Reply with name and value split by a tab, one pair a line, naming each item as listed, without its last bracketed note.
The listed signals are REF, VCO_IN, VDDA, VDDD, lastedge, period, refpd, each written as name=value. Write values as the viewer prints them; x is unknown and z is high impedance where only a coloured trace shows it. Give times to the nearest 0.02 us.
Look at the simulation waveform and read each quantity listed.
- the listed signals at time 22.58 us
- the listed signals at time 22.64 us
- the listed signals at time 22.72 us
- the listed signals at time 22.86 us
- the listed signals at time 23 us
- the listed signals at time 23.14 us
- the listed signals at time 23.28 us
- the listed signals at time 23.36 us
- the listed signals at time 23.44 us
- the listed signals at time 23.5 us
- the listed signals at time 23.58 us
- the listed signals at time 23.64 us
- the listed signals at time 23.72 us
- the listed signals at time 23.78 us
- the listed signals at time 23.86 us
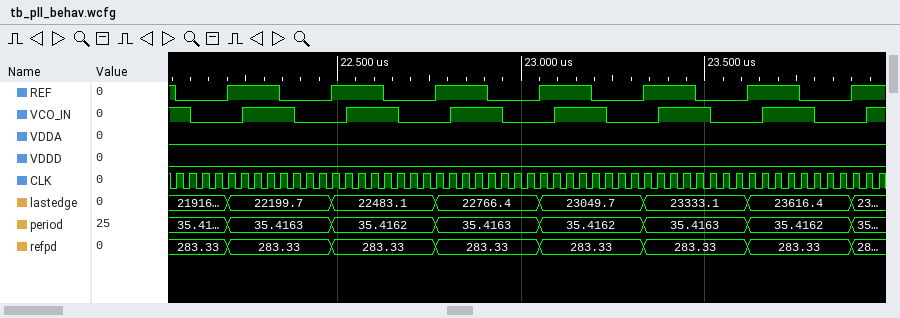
the listed signals at time 22.58 us	REF=1, VCO_IN=1, VDDA=0, VDDD=0, lastedge=22483.1, period=35.4162, refpd=283.33
the listed signals at time 22.64 us	REF=0, VCO_IN=1, VDDA=0, VDDD=0, lastedge=22483.1, period=35.4162, refpd=283.33
the listed signals at time 22.72 us	REF=0, VCO_IN=0, VDDA=0, VDDD=0, lastedge=22483.1, period=35.4162, refpd=283.33
the listed signals at time 22.86 us	REF=1, VCO_IN=1, VDDA=0, VDDD=0, lastedge=22766.4, period=35.4163, refpd=283.33
the listed signals at time 23 us	REF=0, VCO_IN=0, VDDA=0, VDDD=0, lastedge=22766.4, period=35.4163, refpd=283.33
the listed signals at time 23.14 us	REF=1, VCO_IN=1, VDDA=0, VDDD=0, lastedge=23049.7, period=35.4162, refpd=283.33
the listed signals at time 23.28 us	REF=0, VCO_IN=0, VDDA=0, VDDD=0, lastedge=23049.7, period=35.4162, refpd=283.33
the listed signals at time 23.36 us	REF=1, VCO_IN=0, VDDA=0, VDDD=0, lastedge=23333.1, period=35.4163, refpd=283.33
the listed signals at time 23.44 us	REF=1, VCO_IN=1, VDDA=0, VDDD=0, lastedge=23333.1, period=35.4163, refpd=283.33
the listed signals at time 23.5 us	REF=0, VCO_IN=1, VDDA=0, VDDD=0, lastedge=23333.1, period=35.4163, refpd=283.33
the listed signals at time 23.58 us	REF=0, VCO_IN=0, VDDA=0, VDDD=0, lastedge=23333.1, period=35.4163, refpd=283.33
the listed signals at time 23.64 us	REF=1, VCO_IN=0, VDDA=0, VDDD=0, lastedge=23616.4, period=35.4162, refpd=283.33
the listed signals at time 23.72 us	REF=1, VCO_IN=1, VDDA=0, VDDD=0, lastedge=23616.4, period=35.4162, refpd=283.33
the listed signals at time 23.78 us	REF=0, VCO_IN=1, VDDA=0, VDDD=0, lastedge=23616.4, period=35.4162, refpd=283.33
the listed signals at time 23.86 us	REF=0, VCO_IN=0, VDDA=0, VDDD=0, lastedge=23616.4, period=35.4162, refpd=283.33
